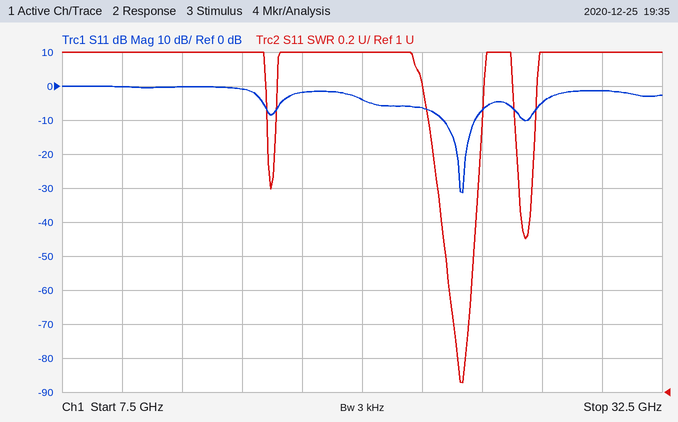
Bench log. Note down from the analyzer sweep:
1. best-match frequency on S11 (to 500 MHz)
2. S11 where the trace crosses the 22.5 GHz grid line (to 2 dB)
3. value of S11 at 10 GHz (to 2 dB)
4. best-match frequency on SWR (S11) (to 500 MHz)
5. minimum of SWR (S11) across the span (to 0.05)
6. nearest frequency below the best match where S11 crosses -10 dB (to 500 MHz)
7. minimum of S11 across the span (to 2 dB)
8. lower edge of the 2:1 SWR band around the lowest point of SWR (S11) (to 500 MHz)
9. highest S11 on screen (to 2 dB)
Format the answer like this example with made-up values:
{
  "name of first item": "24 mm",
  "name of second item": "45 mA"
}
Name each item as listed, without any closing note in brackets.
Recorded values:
{
  "best-match frequency on S11": "24.0 GHz",
  "S11 where the trace crosses the 22.5 GHz grid line": "-6 dB",
  "value of S11 at 10 GHz": "0 dB",
  "best-match frequency on SWR (S11)": "24.0 GHz",
  "minimum of SWR (S11) across the span": "1.05",
  "nearest frequency below the best match where S11 crosses -10 dB": "23.5 GHz",
  "minimum of S11 across the span": "-32 dB",
  "lower edge of the 2:1 SWR band around the lowest point of SWR (S11)": "23.5 GHz",
  "highest S11 on screen": "0 dB"
}
